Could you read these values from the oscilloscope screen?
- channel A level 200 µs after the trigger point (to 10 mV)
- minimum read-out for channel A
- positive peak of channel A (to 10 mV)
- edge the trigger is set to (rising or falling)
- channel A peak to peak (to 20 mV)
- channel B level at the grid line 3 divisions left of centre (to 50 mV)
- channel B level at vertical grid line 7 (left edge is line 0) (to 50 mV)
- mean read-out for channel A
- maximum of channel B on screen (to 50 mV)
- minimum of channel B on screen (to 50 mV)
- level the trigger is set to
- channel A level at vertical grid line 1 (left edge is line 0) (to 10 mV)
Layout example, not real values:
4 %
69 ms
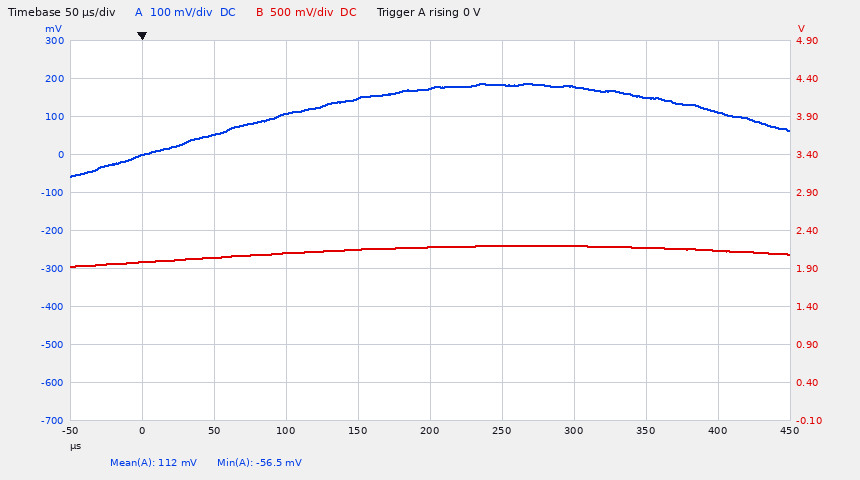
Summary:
170 mV
-56.5 mV
190 mV
rising
240 mV
2.05 V
2.20 V
112 mV
2.20 V
1.95 V
0 V
0 mV
